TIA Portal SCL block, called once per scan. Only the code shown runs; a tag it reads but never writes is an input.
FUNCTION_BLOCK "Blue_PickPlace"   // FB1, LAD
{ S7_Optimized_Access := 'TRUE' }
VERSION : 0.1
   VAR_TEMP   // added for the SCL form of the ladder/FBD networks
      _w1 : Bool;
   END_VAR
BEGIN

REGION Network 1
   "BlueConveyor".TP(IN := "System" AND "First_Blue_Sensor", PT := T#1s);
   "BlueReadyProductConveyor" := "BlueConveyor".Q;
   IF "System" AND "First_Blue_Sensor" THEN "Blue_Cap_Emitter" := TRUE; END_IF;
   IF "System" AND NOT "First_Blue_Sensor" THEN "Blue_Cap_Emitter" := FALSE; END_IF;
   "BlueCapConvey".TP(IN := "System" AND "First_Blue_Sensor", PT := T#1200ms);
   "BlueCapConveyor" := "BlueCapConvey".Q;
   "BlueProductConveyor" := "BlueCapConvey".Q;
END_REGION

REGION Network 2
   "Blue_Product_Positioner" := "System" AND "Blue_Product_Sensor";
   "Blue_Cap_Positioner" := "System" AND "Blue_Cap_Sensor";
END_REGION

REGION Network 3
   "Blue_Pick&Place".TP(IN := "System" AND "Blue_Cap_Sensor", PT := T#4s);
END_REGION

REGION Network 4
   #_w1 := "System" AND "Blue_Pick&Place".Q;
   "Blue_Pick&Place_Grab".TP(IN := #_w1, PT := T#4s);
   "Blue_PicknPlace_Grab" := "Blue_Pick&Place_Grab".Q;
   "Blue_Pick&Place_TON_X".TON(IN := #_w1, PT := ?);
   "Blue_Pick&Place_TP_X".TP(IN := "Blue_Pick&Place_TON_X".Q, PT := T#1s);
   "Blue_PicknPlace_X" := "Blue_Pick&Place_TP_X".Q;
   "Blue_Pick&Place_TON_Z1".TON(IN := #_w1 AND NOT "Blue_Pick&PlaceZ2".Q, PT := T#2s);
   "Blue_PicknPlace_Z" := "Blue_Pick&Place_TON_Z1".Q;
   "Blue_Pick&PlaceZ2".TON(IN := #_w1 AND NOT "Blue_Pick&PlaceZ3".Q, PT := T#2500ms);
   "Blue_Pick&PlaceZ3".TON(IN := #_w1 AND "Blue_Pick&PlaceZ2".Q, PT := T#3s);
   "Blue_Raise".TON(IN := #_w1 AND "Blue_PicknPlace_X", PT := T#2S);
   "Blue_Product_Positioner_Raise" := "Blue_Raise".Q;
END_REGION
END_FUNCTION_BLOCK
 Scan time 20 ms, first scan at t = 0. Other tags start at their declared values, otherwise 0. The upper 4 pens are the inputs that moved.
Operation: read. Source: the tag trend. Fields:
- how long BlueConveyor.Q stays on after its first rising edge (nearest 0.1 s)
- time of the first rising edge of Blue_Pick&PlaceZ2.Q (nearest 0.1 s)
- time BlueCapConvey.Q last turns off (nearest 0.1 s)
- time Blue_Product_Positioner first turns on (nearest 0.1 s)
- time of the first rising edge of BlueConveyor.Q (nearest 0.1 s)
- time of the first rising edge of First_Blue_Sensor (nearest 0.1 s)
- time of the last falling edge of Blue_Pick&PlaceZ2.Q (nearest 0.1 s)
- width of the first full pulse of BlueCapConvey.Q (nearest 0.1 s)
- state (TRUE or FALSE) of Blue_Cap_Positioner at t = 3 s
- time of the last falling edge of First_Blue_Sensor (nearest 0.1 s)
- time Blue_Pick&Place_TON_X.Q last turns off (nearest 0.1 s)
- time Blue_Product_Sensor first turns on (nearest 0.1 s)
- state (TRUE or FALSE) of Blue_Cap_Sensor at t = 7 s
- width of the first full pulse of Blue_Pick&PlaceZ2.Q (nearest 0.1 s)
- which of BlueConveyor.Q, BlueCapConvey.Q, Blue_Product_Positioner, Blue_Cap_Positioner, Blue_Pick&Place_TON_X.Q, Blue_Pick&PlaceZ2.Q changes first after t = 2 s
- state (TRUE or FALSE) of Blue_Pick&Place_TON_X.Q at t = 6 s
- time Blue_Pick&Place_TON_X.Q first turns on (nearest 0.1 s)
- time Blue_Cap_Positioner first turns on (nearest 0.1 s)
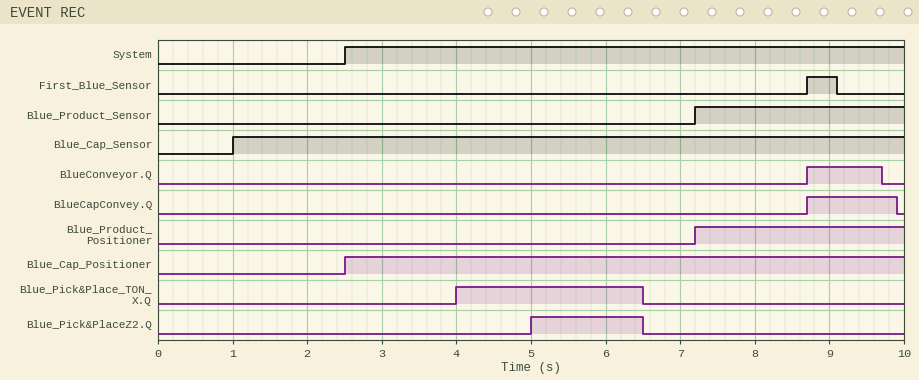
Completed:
1.0 s
5.0 s
9.9 s
7.2 s
8.7 s
8.7 s
6.5 s
1.2 s
TRUE
9.1 s
6.5 s
7.2 s
TRUE
1.5 s
Blue_Cap_Positioner
TRUE
4.0 s
2.5 s
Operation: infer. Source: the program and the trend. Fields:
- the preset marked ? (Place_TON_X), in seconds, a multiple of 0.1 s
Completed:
1.5 s
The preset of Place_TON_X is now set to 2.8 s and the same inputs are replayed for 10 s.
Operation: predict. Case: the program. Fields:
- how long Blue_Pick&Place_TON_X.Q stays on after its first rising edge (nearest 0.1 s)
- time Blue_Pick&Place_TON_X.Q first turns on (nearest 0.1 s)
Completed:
1.2 s
5.3 s
